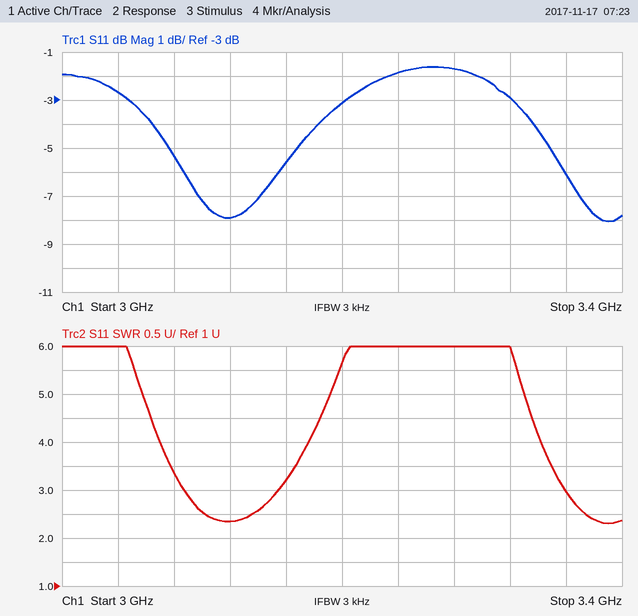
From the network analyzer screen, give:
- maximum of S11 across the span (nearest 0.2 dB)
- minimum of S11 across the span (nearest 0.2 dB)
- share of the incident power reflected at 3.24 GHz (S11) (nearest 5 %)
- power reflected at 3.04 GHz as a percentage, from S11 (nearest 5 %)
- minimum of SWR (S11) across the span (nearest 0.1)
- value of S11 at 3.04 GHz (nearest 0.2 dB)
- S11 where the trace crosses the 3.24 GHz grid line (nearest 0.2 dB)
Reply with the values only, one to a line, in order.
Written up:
-1.6 dB
-8.0 dB
65 %
55 %
2.3
-2.6 dB
-1.8 dB
